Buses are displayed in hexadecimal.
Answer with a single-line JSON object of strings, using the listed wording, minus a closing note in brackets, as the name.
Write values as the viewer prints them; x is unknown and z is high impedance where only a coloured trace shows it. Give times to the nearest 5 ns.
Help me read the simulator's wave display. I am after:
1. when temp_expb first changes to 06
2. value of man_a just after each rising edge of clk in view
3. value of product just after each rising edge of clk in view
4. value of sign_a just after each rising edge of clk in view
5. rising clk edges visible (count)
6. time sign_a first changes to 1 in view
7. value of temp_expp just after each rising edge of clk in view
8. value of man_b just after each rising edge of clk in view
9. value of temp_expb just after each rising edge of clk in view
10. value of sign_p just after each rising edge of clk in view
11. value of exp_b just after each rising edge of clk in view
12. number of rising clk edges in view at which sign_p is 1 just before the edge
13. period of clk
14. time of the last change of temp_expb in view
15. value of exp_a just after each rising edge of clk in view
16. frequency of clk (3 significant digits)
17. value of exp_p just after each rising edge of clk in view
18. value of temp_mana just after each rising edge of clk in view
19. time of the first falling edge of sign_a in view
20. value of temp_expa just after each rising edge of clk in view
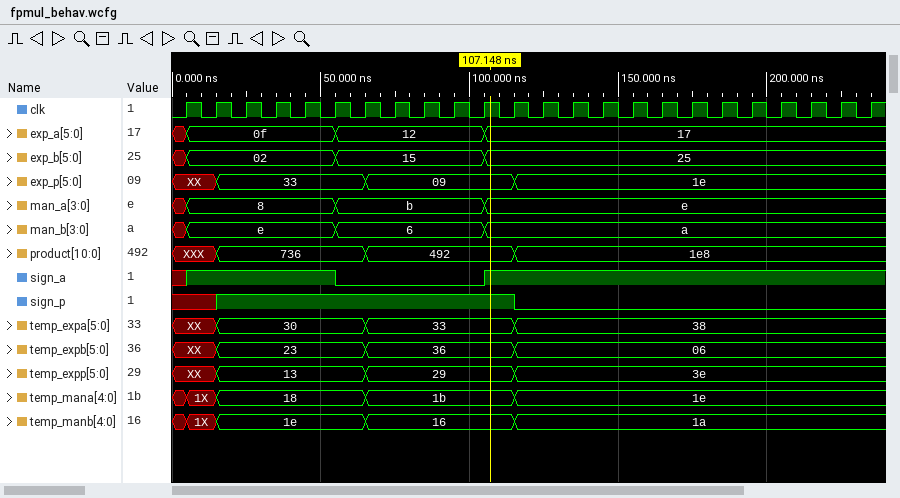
{"when temp_expb first changes to 06": "115 ns", "value of man_a just after each rising edge of clk in view": "8, 8, 8, 8, 8, b, b, b, b, b, e, e, e, e, e, e, e, e, e, e, e, e, e, e", "value of product just after each rising edge of clk in view": "XXX, 736, 736, 736, 736, 736, 492, 492, 492, 492, 492, 1e8, 1e8, 1e8, 1e8, 1e8, 1e8, 1e8, 1e8, 1e8, 1e8, 1e8, 1e8, 1e8", "value of sign_a just after each rising edge of clk in view": "1 1 1 1 1 0 0 0 0 0 1 1 1 1 1 1 1 1 1 1 1 1 1 1", "rising clk edges visible": "24", "time sign_a first changes to 1 in view": "5 ns", "value of temp_expp just after each rising edge of clk in view": "XX, 13, 13, 13, 13, 13, 29, 29, 29, 29, 29, 3e, 3e, 3e, 3e, 3e, 3e, 3e, 3e, 3e, 3e, 3e, 3e, 3e", "value of man_b just after each rising edge of clk in view": "e, e, e, e, e, 6, 6, 6, 6, 6, a, a, a, a, a, a, a, a, a, a, a, a, a, a", "value of temp_expb just after each rising edge of clk in view": "XX, 23, 23, 23, 23, 23, 36, 36, 36, 36, 36, 06, 06, 06, 06, 06, 06, 06, 06, 06, 06, 06, 06, 06", "value of sign_p just after each rising edge of clk in view": "x 1 1 1 1 1 1 1 1 1 1 0 0 0 0 0 0 0 0 0 0 0 0 0", "value of exp_b just after each rising edge of clk in view": "02, 02, 02, 02, 02, 15, 15, 15, 15, 15, 25, 25, 25, 25, 25, 25, 25, 25, 25, 25, 25, 25, 25, 25", "number of rising clk edges in view at which sign_p is 1 just before the edge": "10", "period of clk": "10 ns", "time of the last change of temp_expb in view": "115 ns", "value of exp_a just after each rising edge of clk in view": "0f, 0f, 0f, 0f, 0f, 12, 12, 12, 12, 12, 17, 17, 17, 17, 17, 17, 17, 17, 17, 17, 17, 17, 17, 17", "frequency of clk": "100 MHz", "value of exp_p just after each rising edge of clk in view": "XX, 33, 33, 33, 33, 33, 09, 09, 09, 09, 09, 1e, 1e, 1e, 1e, 1e, 1e, 1e, 1e, 1e, 1e, 1e, 1e, 1e", "value of temp_mana just after each rising edge of clk in view": "1X, 18, 18, 18, 18, 18, 1b, 1b, 1b, 1b, 1b, 1e, 1e, 1e, 1e, 1e, 1e, 1e, 1e, 1e, 1e, 1e, 1e, 1e", "time of the first falling edge of sign_a in view": "55 ns", "value of temp_expa just after each rising edge of clk in view": "XX, 30, 30, 30, 30, 30, 33, 33, 33, 33, 33, 38, 38, 38, 38, 38, 38, 38, 38, 38, 38, 38, 38, 38"}
